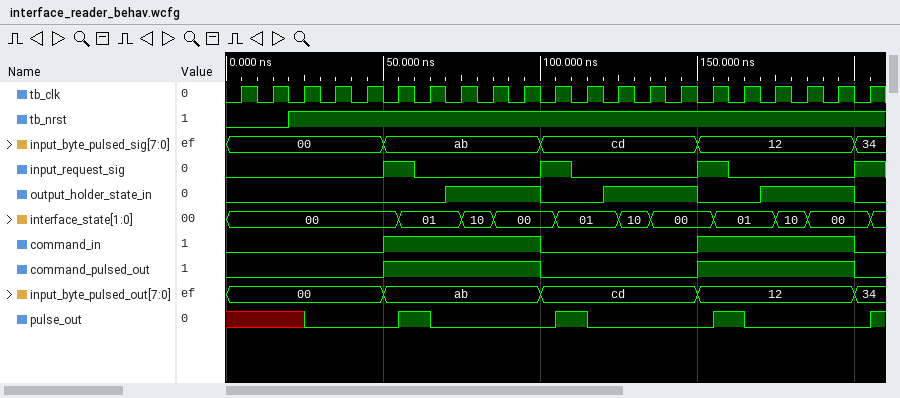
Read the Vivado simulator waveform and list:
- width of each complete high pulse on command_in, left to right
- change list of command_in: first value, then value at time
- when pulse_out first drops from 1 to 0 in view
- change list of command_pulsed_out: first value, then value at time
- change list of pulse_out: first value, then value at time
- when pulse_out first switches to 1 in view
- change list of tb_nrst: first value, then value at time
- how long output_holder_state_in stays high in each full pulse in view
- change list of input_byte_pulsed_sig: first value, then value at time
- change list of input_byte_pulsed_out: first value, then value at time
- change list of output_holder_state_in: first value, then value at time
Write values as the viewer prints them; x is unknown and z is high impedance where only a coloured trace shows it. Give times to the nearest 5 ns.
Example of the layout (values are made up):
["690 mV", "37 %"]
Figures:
["50 ns, 50 ns", "0, 1 at 50 ns, 0 at 100 ns, 1 at 150 ns, 0 at 200 ns", "65 ns", "0, 1 at 50 ns, 0 at 100 ns, 1 at 150 ns, 0 at 200 ns", "x, 0 at 25 ns, 1 at 55 ns, 0 at 65 ns, 1 at 105 ns, 0 at 115 ns, 1 at 155 ns, 0 at 165 ns, 1 at 205 ns", "55 ns", "0, 1 at 20 ns", "30 ns, 30 ns, 30 ns", "00, ab at 50 ns, cd at 100 ns, 12 at 150 ns, 34 at 200 ns", "00, ab at 50 ns, cd at 100 ns, 12 at 150 ns, 34 at 200 ns", "0, 1 at 70 ns, 0 at 100 ns, 1 at 120 ns, 0 at 150 ns, 1 at 170 ns, 0 at 200 ns"]
